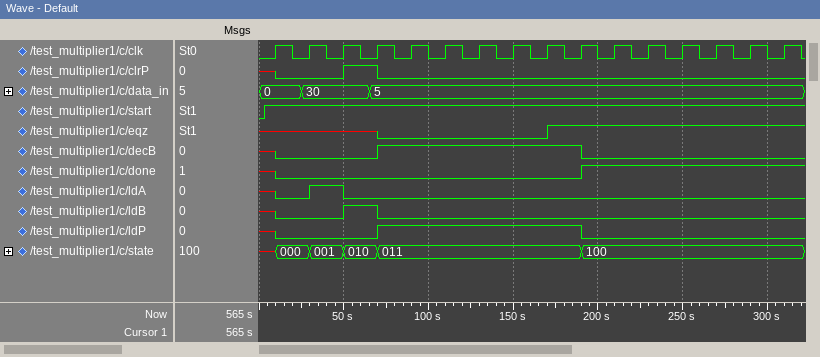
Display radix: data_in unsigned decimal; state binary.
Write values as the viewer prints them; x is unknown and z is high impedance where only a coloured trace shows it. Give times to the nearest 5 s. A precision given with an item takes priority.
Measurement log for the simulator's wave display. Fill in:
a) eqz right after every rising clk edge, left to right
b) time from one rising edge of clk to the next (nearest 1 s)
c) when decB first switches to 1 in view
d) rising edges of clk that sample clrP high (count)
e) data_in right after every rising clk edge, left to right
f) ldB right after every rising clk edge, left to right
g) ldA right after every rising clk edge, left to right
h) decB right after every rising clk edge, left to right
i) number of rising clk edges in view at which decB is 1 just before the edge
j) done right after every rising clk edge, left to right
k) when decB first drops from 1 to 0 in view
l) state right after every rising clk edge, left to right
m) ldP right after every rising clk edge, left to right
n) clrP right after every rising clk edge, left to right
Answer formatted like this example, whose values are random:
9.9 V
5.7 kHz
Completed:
x x x 0 0 0 0 0 1 1 1 1 1 1 1 1
20 s
70 s
1
0, 30, 30, 5, 5, 5, 5, 5, 5, 5, 5, 5, 5, 5, 5, 5
0 0 1 0 0 0 0 0 0 0 0 0 0 0 0 0
0 1 0 0 0 0 0 0 0 0 0 0 0 0 0 0
0 0 0 1 1 1 1 1 1 0 0 0 0 0 0 0
6
0 0 0 0 0 0 0 0 0 1 1 1 1 1 1 1
190 s
000, 001, 010, 011, 011, 011, 011, 011, 011, 100, 100, 100, 100, 100, 100, 100
0 0 0 1 1 1 1 1 1 0 0 0 0 0 0 0
0 0 1 0 0 0 0 0 0 0 0 0 0 0 0 0
